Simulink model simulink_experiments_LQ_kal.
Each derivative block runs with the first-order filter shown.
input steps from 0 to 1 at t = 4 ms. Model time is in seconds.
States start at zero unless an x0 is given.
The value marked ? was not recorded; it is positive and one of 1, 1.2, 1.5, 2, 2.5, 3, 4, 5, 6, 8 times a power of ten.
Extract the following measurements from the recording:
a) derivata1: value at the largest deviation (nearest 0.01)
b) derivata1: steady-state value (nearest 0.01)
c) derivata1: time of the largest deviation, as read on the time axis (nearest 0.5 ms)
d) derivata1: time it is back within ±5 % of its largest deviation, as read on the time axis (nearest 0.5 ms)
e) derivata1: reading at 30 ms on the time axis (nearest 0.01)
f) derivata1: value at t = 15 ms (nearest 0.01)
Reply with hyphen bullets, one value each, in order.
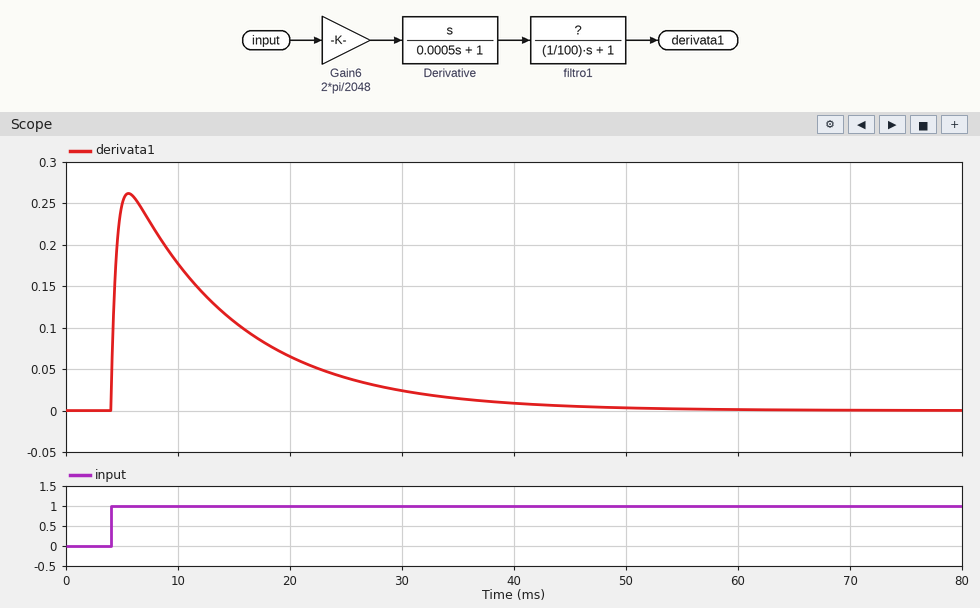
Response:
- 0.26
- 0.00
- 5.5 ms
- 36.0 ms
- 0.02
- 0.11
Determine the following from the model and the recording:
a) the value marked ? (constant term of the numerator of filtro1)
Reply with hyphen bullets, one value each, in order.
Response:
- 1
